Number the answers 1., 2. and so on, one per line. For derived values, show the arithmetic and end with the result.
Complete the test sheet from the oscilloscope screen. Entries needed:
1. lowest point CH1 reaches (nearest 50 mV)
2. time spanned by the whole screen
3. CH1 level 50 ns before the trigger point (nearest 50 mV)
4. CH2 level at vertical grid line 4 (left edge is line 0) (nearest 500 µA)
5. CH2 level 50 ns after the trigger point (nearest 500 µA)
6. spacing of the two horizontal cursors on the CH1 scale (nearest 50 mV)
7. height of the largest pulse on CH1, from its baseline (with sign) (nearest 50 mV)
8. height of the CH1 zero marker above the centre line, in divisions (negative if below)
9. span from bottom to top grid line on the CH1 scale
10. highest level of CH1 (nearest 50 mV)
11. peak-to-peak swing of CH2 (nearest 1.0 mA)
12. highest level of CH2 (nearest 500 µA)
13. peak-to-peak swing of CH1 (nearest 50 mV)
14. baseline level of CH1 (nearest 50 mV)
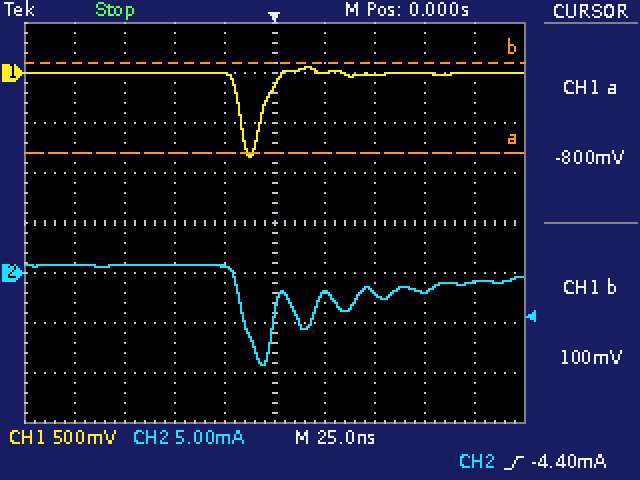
1. -850 mV
2. 250 ns
3. 0 mV
4. 500 µA
5. -2.0 mA
6. 900 mV
7. -850 mV − (0 mV) = -850 mV
8. +3.0 div
9. 4 V
10. 50 mV
11. 10.0 mA
12. 1.0 mA
13. 50 mV − (-850 mV) = 900 mV
14. 0 mV
